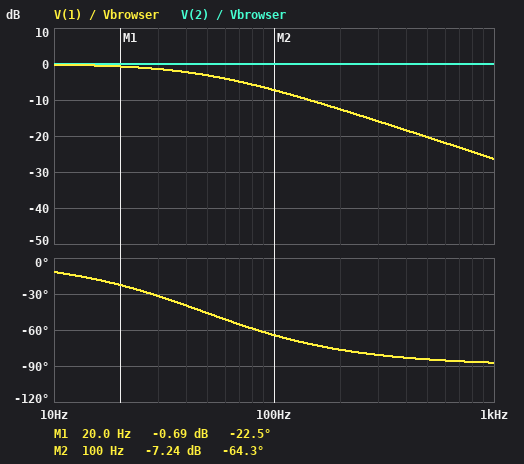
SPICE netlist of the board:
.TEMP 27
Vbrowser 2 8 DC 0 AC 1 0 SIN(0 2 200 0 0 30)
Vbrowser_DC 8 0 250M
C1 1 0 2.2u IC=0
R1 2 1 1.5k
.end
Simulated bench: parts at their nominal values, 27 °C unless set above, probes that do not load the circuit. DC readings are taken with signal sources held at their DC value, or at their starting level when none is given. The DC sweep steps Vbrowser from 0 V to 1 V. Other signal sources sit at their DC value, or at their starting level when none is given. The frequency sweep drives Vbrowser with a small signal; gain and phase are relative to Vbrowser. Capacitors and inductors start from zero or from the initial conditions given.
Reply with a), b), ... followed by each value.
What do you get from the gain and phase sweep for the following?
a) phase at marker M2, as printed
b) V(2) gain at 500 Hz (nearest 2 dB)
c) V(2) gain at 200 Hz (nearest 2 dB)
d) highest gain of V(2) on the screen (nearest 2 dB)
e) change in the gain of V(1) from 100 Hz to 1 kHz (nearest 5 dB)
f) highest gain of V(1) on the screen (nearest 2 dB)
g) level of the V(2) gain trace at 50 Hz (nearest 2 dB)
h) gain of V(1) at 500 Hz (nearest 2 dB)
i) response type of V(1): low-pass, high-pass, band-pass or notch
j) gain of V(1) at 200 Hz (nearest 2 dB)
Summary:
a) -64.3 deg
b) 0 dB
c) 0 dB
d) 0 dB
e) -20 dB
f) 0 dB
g) 0 dB
h) -20 dB
i) low-pass
j) -12 dB
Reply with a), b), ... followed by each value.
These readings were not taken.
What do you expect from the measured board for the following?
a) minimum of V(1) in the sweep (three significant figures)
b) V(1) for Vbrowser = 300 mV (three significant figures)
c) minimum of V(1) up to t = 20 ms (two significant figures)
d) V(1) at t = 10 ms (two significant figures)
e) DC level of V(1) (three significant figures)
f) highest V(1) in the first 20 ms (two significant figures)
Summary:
a) 250 mV
b) 550 mV
c) -220 mV
d) -85 mV
e) 250 mV
f) 770 mV
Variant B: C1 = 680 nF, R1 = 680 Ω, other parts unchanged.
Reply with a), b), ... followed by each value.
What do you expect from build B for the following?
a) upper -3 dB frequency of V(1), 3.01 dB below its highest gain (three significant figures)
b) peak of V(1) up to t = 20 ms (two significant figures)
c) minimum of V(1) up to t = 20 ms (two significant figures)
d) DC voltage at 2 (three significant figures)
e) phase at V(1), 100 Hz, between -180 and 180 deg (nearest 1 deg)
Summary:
a) 344 Hz
b) 2.0 V
c) -1.5 V
d) 250 mV
e) -16 deg
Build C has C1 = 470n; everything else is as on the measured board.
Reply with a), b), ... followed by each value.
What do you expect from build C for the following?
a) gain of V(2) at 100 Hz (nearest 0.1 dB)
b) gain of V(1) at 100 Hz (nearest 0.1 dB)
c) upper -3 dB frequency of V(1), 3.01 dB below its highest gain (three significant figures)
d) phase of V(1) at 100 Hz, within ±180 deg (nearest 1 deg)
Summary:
a) 0 dB
b) -0.8 dB
c) 226 Hz
d) -24 deg
